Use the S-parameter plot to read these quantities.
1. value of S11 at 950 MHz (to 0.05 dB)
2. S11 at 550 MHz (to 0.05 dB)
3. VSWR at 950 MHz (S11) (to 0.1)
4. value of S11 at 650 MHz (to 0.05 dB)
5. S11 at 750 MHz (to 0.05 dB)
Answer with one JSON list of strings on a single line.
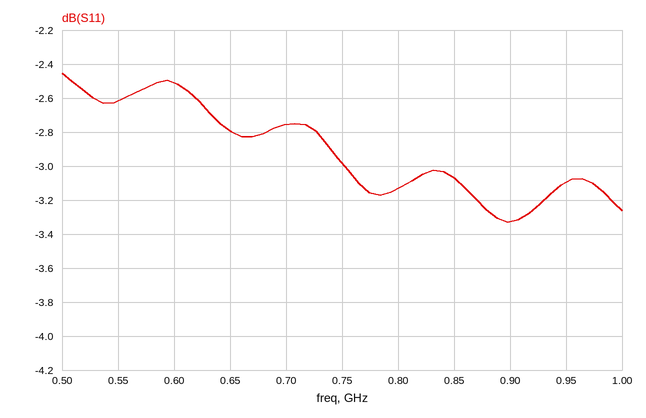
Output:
["-3.10 dB", "-2.60 dB", "5.7", "-2.80 dB", "-3.00 dB"]
